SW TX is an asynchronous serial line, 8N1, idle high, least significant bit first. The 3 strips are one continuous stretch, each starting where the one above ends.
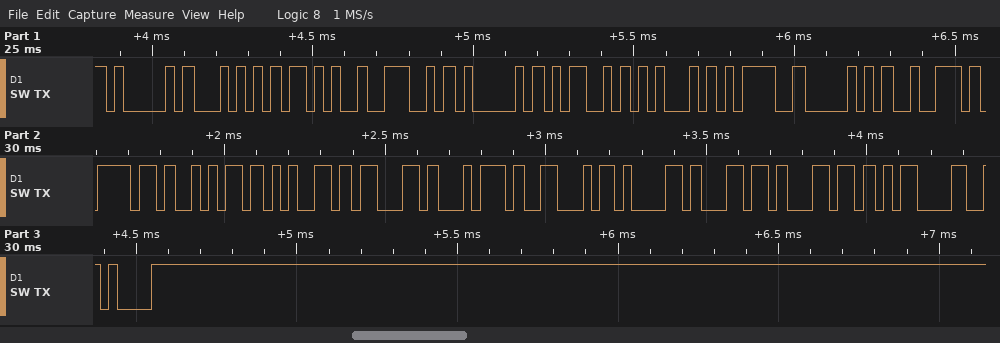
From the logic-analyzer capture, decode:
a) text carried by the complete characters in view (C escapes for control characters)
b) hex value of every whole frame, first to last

"AT+NAME=ProjectFall\r\n"
41 54 2B 4E 41 4D 45 3D 50 72 6F 6A 65 63 74 46 61 6C 6C 0D 0A
